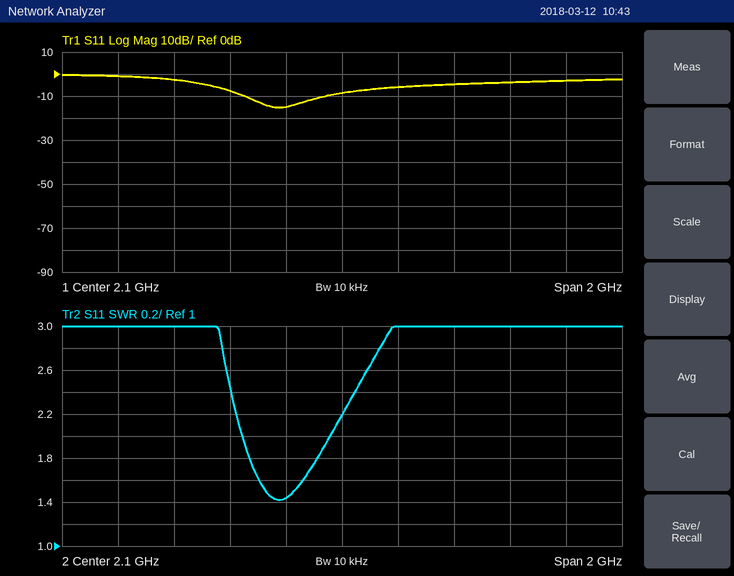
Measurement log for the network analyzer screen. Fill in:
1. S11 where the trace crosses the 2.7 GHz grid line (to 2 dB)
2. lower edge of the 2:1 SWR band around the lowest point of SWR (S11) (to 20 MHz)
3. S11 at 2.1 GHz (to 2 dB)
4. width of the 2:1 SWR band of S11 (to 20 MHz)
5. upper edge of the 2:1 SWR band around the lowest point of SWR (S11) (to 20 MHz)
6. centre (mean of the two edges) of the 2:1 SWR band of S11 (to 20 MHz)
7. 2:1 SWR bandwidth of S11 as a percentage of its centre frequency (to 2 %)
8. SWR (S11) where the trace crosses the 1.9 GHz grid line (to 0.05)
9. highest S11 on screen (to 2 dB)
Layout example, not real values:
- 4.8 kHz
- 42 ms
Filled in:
- -4 dB
- 1.74 GHz
- -8 dB
- 320 MHz
- 2.06 GHz
- 1.90 GHz
- 16 %
- 1.45
- 0 dB
